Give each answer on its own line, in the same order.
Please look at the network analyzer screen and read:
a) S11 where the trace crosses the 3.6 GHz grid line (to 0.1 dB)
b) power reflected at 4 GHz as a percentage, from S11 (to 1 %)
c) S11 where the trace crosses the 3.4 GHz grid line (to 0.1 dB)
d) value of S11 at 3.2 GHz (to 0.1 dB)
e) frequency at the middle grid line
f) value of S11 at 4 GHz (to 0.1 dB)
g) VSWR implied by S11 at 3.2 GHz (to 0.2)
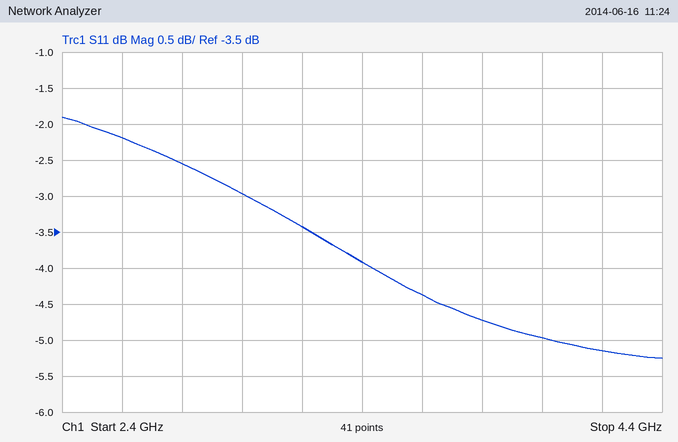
-4.4 dB
32 %
-3.9 dB
-3.4 dB
3.4 GHz
-5.0 dB
5.2
